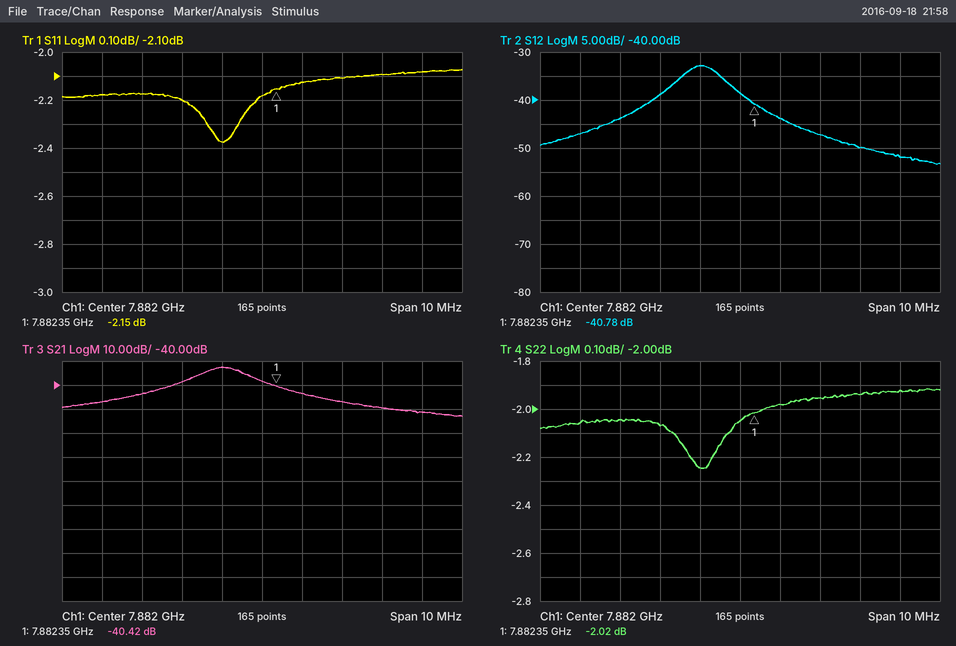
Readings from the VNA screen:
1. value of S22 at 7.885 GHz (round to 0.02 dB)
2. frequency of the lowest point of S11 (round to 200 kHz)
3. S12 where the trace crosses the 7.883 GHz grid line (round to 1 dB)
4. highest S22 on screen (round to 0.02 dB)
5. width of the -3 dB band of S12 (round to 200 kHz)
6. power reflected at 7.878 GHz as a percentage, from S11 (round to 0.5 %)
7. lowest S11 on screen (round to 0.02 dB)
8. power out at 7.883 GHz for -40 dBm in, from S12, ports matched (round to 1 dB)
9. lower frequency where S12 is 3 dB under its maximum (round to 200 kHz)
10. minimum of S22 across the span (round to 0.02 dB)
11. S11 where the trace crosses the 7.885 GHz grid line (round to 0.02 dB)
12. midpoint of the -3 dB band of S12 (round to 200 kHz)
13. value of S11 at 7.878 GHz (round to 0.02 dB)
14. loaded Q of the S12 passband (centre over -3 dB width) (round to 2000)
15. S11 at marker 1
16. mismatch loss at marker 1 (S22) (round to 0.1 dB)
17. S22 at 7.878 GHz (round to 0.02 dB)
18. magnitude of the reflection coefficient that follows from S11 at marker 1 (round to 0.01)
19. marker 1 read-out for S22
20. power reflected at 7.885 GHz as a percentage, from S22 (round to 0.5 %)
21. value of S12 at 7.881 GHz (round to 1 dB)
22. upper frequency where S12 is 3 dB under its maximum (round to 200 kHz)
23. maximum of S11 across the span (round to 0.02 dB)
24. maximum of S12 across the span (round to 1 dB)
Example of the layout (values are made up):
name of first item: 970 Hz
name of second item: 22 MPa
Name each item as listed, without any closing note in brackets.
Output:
value of S22 at 7.885 GHz: -1.94 dB
frequency of the lowest point of S11: 7.8810 GHz
S12 where the trace crosses the 7.883 GHz grid line: -44 dB
highest S22 on screen: -1.92 dB
width of the -3 dB band of S12: 1.2 MHz
power reflected at 7.878 GHz as a percentage, from S11: 60.5 %
lowest S11 on screen: -2.38 dB
power out at 7.883 GHz for -40 dBm in, from S12, ports matched: -84 dBm
lower frequency where S12 is 3 dB under its maximum: 7.8804 GHz
minimum of S22 across the span: -2.24 dB
S11 where the trace crosses the 7.885 GHz grid line: -2.10 dB
midpoint of the -3 dB band of S12: 7.8810 GHz
value of S11 at 7.878 GHz: -2.18 dB
loaded Q of the S12 passband (centre over -3 dB width): 6000
S11 at marker 1: -2.15 dB
mismatch loss at marker 1 (S22): 4.3 dB
S22 at 7.878 GHz: -2.06 dB
magnitude of the reflection coefficient that follows from S11 at marker 1: 0.78
marker 1 read-out for S22: -2.02 dB
power reflected at 7.885 GHz as a percentage, from S22: 64.0 %
value of S12 at 7.881 GHz: -33 dB
upper frequency where S12 is 3 dB under its maximum: 7.8816 GHz
maximum of S11 across the span: -2.08 dB
maximum of S12 across the span: -33 dB
